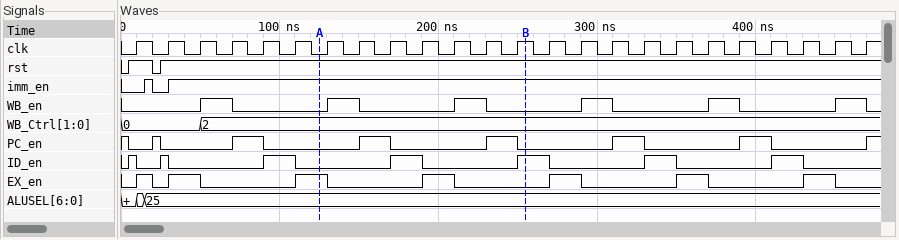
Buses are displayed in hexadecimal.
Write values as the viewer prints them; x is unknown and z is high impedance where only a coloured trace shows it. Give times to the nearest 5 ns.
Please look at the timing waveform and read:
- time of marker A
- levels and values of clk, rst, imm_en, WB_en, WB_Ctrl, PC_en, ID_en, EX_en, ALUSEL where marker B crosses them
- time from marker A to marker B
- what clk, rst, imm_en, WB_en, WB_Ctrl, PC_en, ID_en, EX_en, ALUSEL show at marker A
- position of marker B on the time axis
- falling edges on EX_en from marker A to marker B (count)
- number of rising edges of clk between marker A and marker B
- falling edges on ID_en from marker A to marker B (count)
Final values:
125 ns
clk=1, rst=1, imm_en=1, WB_en=0, WB_Ctrl=2, PC_en=0, ID_en=1, EX_en=0, ALUSEL=25
130 ns
clk=0, rst=1, imm_en=1, WB_en=0, WB_Ctrl=2, PC_en=0, ID_en=0, EX_en=1, ALUSEL=25
255 ns
2
7
1
